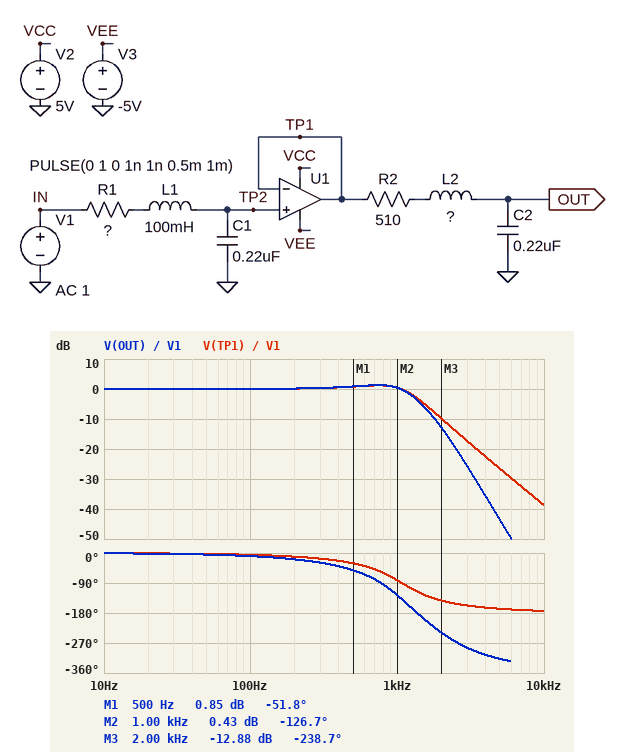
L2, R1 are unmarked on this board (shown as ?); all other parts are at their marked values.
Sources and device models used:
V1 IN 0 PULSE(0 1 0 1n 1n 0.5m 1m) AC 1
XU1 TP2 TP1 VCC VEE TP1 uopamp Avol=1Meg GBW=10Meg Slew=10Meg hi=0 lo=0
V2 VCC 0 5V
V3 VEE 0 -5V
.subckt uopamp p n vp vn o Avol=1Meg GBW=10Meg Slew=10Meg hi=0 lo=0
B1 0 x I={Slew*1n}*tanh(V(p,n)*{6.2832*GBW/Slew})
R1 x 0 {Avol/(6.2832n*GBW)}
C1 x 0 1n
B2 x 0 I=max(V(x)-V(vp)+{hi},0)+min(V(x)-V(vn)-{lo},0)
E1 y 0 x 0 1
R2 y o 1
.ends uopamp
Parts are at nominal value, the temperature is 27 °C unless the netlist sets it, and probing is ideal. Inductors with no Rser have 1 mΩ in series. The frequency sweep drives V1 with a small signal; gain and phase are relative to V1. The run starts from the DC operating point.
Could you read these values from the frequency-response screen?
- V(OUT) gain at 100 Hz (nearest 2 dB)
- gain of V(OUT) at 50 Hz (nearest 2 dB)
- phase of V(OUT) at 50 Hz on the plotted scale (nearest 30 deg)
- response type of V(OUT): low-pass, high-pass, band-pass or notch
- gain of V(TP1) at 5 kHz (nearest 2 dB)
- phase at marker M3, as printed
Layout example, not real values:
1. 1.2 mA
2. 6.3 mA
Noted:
1. 0 dB
2. 0 dB
3. 0 deg
4. low-pass
5. -26 dB
6. -238.7 deg
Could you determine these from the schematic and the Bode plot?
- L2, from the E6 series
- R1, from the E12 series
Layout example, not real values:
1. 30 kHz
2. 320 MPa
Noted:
1. 33 mH
2. 680 Ω
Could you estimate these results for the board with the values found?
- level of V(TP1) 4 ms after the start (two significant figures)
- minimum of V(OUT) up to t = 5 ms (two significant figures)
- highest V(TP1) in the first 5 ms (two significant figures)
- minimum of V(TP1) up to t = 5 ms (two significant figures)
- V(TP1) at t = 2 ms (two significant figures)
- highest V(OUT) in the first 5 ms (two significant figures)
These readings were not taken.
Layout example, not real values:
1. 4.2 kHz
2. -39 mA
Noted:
1. -180 mV
2. -170 mV
3. 1.2 V
4. -180 mV
5. -180 mV
6. 1.2 V
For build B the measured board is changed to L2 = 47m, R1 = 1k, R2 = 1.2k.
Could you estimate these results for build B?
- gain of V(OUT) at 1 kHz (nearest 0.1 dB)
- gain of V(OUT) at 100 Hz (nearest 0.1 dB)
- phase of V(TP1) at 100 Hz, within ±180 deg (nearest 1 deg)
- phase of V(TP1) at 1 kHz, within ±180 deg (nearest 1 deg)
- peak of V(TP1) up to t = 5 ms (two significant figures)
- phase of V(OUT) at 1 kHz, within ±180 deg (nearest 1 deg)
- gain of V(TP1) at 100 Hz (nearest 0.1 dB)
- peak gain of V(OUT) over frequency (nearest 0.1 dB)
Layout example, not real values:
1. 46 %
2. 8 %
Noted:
1. -7.8 dB
2. -0.1 dB
3. -8 deg
4. -85 deg
5. 990 mV
6. -155 deg
7. 0 dB
8. 0 dB
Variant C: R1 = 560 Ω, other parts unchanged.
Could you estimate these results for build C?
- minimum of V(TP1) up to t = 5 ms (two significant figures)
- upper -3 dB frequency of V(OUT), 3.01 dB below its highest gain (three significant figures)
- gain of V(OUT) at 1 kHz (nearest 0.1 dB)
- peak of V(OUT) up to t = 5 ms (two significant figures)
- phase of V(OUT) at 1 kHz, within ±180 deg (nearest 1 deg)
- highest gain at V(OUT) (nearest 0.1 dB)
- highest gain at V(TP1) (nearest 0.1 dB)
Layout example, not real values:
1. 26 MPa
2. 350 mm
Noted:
1. -310 mV
2. 1.24 kHz
3. 2.1 dB
4. 1.3 V
5. -125 deg
6. 2.5 dB
7. 2.4 dB
